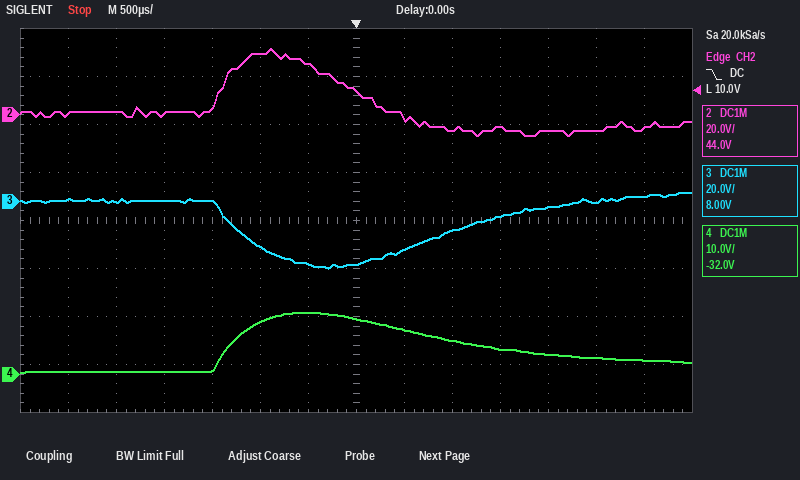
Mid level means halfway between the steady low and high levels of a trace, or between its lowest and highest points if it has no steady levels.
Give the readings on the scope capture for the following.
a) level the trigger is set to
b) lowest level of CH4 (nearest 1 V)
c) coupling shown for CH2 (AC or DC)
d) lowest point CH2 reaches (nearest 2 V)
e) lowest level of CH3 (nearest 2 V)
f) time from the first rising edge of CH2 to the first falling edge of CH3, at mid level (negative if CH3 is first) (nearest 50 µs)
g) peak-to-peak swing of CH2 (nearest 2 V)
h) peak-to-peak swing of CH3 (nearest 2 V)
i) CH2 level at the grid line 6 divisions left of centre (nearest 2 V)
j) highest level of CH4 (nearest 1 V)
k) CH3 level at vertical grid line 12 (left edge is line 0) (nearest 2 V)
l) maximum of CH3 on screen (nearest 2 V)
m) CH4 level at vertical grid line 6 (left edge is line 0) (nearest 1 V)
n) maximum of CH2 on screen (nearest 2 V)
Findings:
10.0 V
0 V
DC
-8 V
-28 V
+200 µs
36 V
32 V
0 V
13 V
0 V
4 V
13 V
28 V
